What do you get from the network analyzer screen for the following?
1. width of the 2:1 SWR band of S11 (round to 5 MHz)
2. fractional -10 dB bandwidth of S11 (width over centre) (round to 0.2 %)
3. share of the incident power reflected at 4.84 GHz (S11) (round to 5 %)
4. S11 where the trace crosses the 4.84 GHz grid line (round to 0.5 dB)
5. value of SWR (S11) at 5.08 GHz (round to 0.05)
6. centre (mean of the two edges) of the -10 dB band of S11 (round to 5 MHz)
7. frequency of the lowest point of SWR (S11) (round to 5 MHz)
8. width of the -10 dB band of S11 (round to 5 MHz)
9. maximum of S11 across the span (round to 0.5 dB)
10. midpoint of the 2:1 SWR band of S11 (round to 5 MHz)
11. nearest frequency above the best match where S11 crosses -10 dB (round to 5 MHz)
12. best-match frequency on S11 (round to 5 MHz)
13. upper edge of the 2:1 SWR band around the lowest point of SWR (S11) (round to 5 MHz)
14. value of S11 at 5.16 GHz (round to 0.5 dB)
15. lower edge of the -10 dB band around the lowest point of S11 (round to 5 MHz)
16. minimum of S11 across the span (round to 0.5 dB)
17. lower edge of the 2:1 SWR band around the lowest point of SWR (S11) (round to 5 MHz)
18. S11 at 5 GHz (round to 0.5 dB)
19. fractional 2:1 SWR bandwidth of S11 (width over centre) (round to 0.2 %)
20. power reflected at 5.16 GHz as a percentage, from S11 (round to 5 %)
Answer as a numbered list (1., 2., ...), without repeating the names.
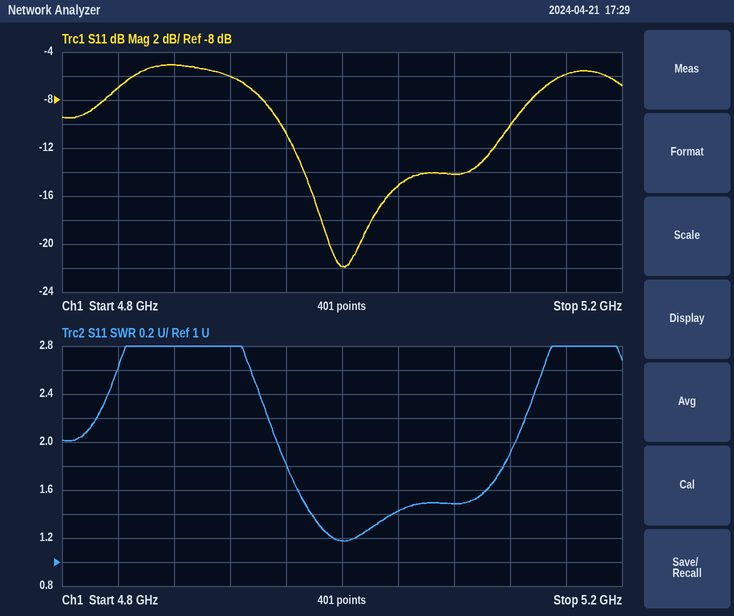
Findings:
1. 170 MHz
2. 3.2 %
3. 20 %
4. -7.0 dB
5. 1.50
6. 5.040 GHz
7. 5.000 GHz
8. 165 MHz
9. -5.0 dB
10. 5.040 GHz
11. 5.120 GHz
12. 5.000 GHz
13. 5.125 GHz
14. -6.0 dB
15. 4.955 GHz
16. -22.0 dB
17. 4.955 GHz
18. -22.0 dB
19. 3.4 %
20. 25 %
